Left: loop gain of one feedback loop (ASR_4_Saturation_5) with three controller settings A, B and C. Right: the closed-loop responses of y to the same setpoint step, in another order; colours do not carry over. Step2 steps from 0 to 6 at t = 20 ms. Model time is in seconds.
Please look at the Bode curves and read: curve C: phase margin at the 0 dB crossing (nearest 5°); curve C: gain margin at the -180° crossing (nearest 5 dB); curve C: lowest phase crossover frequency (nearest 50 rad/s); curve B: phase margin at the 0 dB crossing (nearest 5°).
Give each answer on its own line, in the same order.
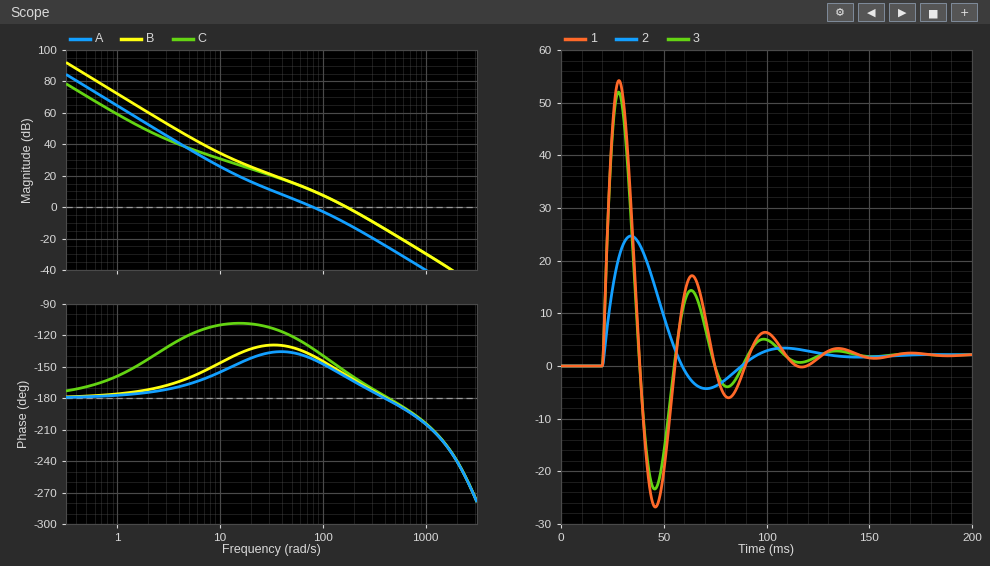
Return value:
25°
15 dB
450 rad/s
20°
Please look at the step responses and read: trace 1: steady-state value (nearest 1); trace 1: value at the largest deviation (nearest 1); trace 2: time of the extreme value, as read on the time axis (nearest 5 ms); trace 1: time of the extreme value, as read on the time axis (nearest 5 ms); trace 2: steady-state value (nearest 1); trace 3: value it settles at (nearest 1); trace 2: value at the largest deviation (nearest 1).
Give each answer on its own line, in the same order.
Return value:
2
54
35 ms
30 ms
2
2
25
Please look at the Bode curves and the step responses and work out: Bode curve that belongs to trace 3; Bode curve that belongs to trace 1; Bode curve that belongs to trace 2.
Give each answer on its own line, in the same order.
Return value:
C
B
A
